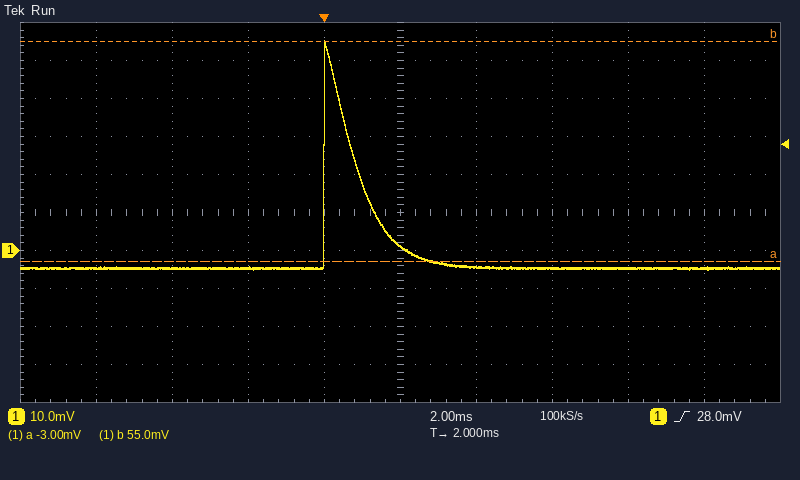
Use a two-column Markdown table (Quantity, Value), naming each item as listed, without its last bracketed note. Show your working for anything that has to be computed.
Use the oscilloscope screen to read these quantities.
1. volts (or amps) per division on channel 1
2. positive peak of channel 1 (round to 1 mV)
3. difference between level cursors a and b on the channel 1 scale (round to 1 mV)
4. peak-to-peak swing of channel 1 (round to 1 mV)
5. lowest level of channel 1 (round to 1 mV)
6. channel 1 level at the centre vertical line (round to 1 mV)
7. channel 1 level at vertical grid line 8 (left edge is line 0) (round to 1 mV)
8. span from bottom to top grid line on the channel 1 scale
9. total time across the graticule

| Quantity | Value |
|---|---|
| volts (or amps) per division on channel 1 | 10 mV |
| positive peak of channel 1 | 55 mV |
| difference between level cursors a and b on the channel 1 scale | 58 mV |
| peak-to-peak swing of channel 1 | 55 mV − (-5 mV) = 60 mV |
| lowest level of channel 1 | -5 mV |
| channel 1 level at the centre vertical line | 1 mV |
| channel 1 level at vertical grid line 8 (left edge is line 0) | -5 mV |
| span from bottom to top grid line on the channel 1 scale | 100 mV |
| total time across the graticule | 20 ms |
